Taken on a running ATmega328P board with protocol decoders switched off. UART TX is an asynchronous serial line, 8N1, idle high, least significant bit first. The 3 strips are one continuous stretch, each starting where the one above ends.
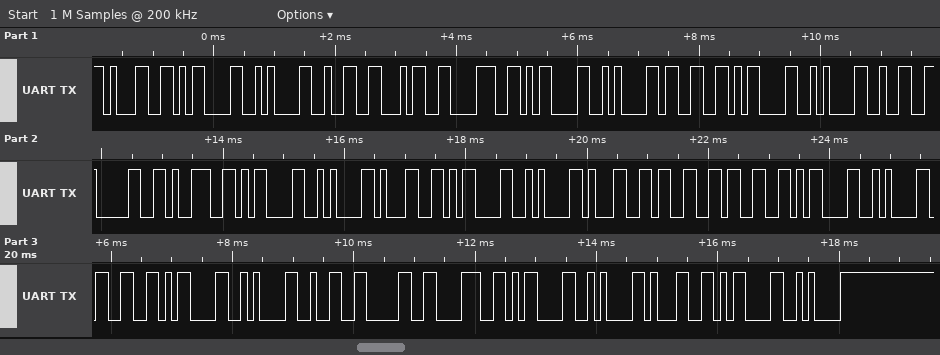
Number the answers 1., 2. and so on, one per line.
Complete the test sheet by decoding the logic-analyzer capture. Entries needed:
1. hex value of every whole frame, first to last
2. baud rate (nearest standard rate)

1. 31 0D 0A 32 34 38 0D 0A 33 0D 0A 32 30 39 0D 0A 31 0D 0A 31 33 33 0D 0A 33 0D 0A 32 30 38 0D 0A 31 0D 0A
2. 9600 baud
